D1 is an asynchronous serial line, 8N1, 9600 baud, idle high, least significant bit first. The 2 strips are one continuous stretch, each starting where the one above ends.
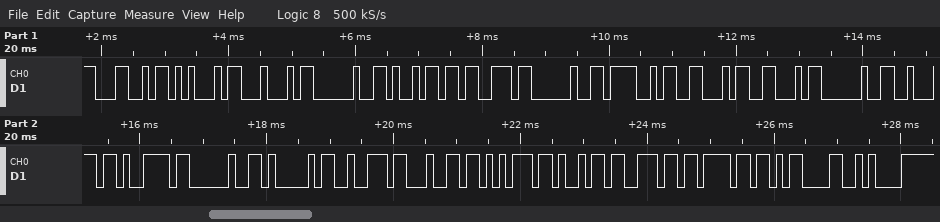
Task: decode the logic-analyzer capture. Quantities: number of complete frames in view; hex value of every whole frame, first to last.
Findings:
23
4C 45 44 20 69 73 20 4F 46 46 20 62 79 20 41 72 64 75 69 6E 6F 0D 0A
